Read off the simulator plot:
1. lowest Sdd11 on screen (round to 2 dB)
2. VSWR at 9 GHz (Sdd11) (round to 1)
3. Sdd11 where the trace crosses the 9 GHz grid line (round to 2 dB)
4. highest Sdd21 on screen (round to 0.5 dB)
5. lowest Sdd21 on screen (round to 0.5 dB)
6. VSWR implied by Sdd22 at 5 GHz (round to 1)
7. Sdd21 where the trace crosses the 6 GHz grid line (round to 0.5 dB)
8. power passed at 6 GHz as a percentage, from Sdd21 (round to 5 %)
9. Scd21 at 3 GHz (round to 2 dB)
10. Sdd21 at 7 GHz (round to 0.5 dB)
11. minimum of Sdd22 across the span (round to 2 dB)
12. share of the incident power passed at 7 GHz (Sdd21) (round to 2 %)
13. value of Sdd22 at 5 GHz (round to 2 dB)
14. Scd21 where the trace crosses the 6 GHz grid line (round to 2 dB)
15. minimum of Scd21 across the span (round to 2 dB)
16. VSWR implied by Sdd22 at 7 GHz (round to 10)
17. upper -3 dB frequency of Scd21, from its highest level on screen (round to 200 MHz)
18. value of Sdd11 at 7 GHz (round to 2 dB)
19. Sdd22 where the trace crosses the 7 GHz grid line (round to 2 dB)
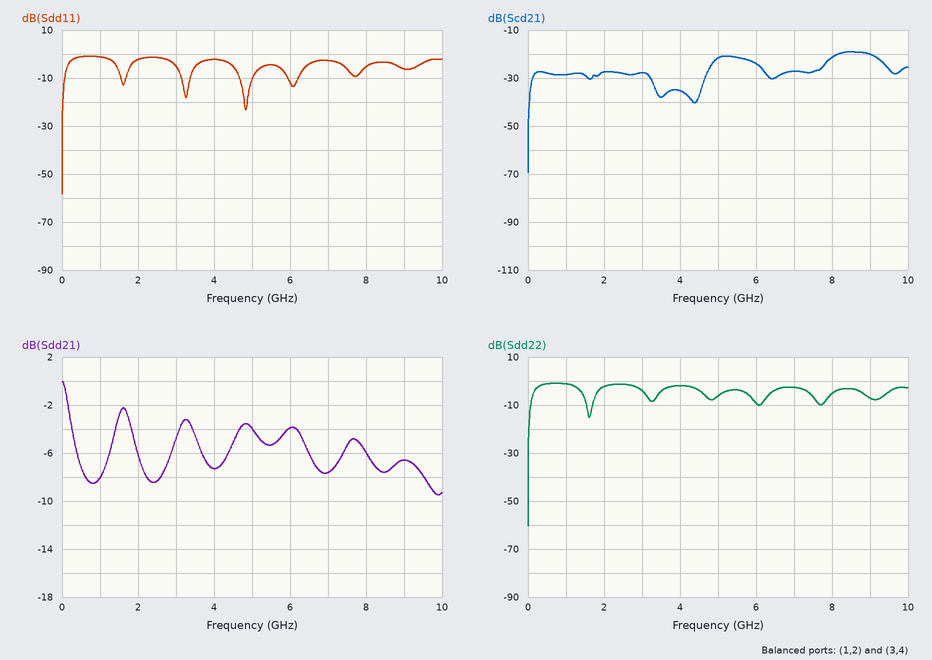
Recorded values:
-58 dB
3
-6 dB
0.0 dB
-9.5 dB
3
-4.0 dB
40 %
-28 dB
-7.5 dB
-60 dB
18 %
-6 dB
-24 dB
-70 dB
10
9.2 GHz
-2 dB
-2 dB
